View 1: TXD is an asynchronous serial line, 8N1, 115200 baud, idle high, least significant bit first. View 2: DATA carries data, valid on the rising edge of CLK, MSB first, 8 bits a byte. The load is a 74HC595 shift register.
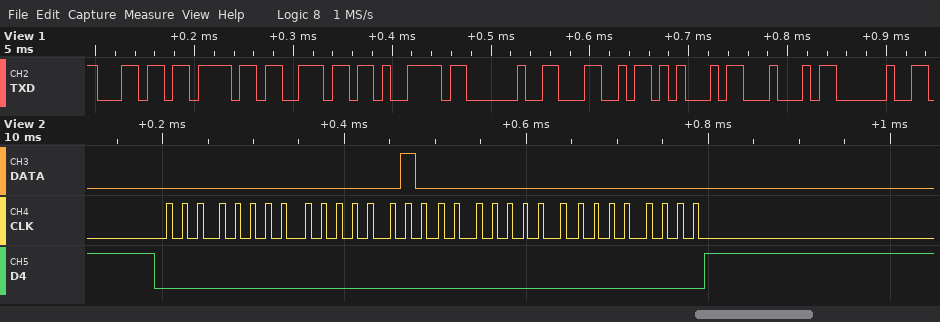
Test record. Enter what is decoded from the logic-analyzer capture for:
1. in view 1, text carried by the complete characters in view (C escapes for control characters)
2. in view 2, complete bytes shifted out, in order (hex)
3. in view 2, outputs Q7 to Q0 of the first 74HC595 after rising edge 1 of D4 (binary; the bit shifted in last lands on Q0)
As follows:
"lony LED "
00 02 00 00
00000000
